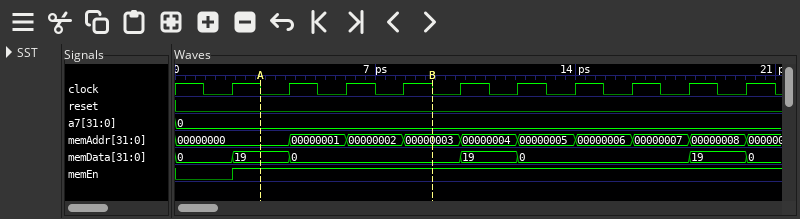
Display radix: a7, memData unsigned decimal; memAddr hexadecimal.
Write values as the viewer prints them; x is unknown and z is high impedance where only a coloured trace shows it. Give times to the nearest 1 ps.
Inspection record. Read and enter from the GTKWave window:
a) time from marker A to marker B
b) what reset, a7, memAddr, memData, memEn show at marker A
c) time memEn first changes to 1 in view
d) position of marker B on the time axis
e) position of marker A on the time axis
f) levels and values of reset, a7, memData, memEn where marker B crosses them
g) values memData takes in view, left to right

6 ps
reset=0, a7=0, memAddr=00000000, memData=19, memEn=1
2 ps
9 ps
3 ps
reset=0, a7=0, memData=0, memEn=1
0, 19, 0, 19, 0, 19, 0
